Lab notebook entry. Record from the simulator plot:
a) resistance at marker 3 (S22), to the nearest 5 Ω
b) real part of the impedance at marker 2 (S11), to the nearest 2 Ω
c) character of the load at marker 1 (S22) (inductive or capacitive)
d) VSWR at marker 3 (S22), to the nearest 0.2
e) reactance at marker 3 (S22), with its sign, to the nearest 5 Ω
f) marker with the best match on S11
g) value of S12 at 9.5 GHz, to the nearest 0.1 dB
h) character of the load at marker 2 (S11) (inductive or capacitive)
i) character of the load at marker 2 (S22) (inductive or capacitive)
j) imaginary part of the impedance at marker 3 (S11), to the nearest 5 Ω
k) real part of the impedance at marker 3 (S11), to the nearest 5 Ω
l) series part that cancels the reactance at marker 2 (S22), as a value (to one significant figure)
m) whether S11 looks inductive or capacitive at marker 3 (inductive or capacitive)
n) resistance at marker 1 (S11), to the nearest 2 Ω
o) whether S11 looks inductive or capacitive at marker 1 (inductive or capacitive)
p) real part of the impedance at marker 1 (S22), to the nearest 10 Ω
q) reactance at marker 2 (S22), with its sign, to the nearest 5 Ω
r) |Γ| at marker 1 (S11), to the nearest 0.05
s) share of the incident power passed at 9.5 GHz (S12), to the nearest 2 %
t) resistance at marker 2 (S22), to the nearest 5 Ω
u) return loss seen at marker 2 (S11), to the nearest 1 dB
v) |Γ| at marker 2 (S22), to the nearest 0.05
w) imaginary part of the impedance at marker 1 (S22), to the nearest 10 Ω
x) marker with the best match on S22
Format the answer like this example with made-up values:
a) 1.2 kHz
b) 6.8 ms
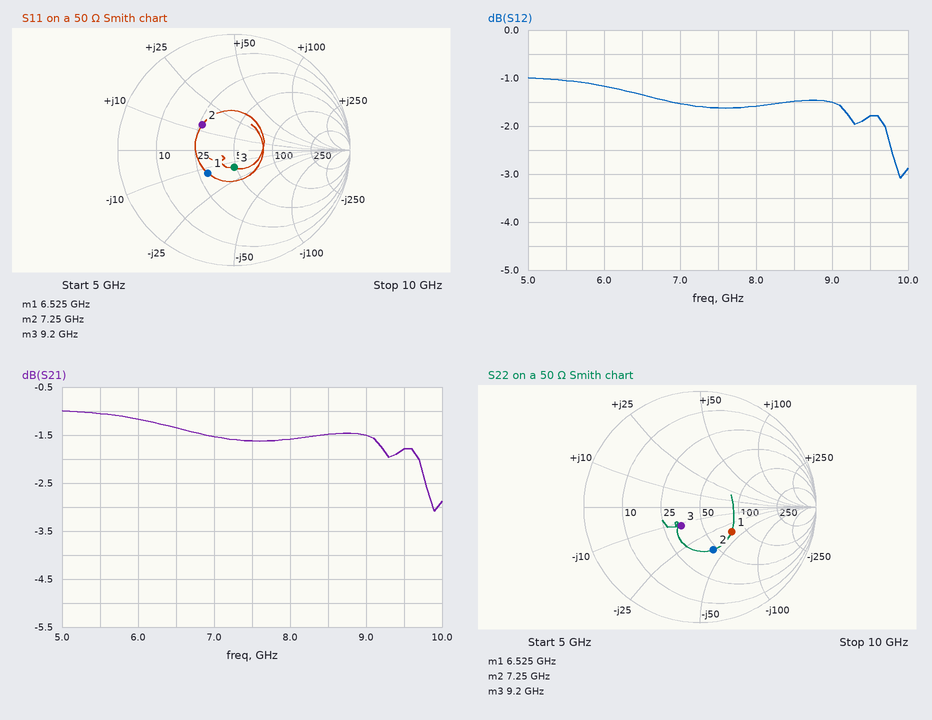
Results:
a) 35 Ω
b) 26 Ω
c) capacitive
d) 1.6
e) -10 Ω
f) marker 3
g) -1.8 dB
h) inductive
i) capacitive
j) -15 Ω
k) 50 Ω
l) 900 pH
m) capacitive
n) 30 Ω
o) capacitive
p) 80 Ω
q) -40 Ω
r) 0.30
s) 66 %
t) 45 Ω
u) 9 dB
v) 0.40
w) -40 Ω
x) marker 3
